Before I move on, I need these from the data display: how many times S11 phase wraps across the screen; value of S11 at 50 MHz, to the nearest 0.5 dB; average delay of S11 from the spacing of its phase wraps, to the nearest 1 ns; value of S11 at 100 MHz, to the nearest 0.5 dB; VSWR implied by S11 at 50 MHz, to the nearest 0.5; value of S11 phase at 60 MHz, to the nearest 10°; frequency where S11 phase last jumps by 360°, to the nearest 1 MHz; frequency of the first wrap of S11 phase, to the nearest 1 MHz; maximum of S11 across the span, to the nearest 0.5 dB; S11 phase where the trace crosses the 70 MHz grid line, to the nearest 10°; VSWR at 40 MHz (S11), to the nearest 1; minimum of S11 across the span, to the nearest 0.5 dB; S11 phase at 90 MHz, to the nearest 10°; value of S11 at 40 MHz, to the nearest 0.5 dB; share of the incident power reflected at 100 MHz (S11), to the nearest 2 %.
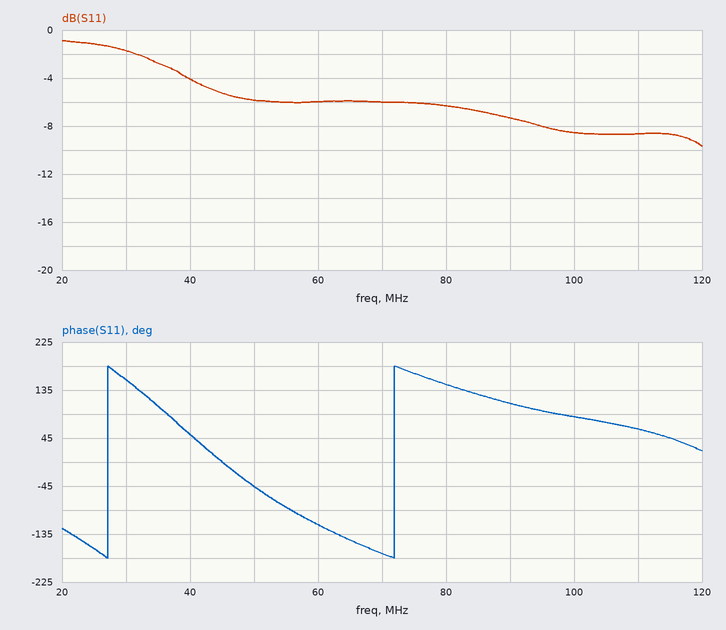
2
-6.0 dB
22 ns
-8.5 dB
3.0
-120°
72 MHz
27 MHz
-1.0 dB
-170°
4
-9.5 dB
110°
-4.0 dB
14 %
